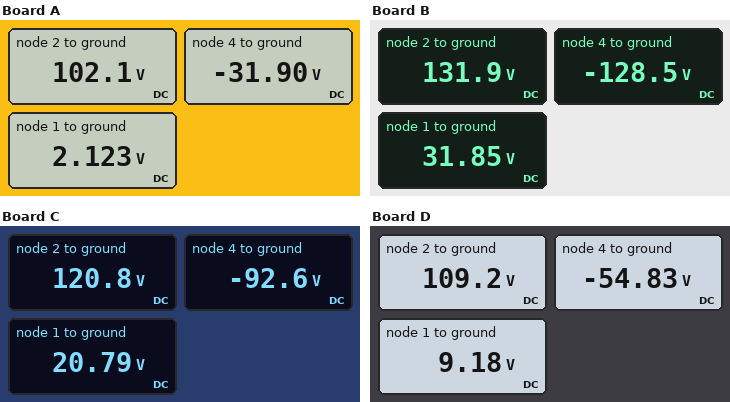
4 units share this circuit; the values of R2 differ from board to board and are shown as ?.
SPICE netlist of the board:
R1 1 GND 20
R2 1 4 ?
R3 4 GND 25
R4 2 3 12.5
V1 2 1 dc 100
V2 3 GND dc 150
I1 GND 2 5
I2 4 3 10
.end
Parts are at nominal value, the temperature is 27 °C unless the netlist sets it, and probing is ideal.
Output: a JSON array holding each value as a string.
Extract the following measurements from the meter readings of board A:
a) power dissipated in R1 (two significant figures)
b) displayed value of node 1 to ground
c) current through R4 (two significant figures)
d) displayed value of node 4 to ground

["230 mW", "2.123 V", "3.8 A", "-31.90 V"]
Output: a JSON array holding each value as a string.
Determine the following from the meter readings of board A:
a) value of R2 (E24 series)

["3.9 Ω"]
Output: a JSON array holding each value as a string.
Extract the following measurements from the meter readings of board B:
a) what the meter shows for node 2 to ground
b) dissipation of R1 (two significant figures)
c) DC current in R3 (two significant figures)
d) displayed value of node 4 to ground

["131.9 V", "51 W", "5.1 A", "-128.5 V"]
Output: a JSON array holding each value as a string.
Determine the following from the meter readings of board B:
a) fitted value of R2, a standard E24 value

["33 Ω"]
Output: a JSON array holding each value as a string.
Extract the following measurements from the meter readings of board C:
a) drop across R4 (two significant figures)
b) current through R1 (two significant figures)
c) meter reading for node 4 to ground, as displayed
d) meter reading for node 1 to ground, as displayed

["29 V", "1.0 A", "-92.6 V", "20.79 V"]
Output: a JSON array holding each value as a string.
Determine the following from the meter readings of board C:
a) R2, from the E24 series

["18 Ω"]
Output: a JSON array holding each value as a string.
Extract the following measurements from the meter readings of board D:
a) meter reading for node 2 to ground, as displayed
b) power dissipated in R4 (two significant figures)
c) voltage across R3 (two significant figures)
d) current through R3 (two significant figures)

["109.2 V", "130 W", "55 V", "2.2 A"]
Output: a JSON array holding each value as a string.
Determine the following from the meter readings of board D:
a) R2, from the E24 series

["8.2 Ω"]
